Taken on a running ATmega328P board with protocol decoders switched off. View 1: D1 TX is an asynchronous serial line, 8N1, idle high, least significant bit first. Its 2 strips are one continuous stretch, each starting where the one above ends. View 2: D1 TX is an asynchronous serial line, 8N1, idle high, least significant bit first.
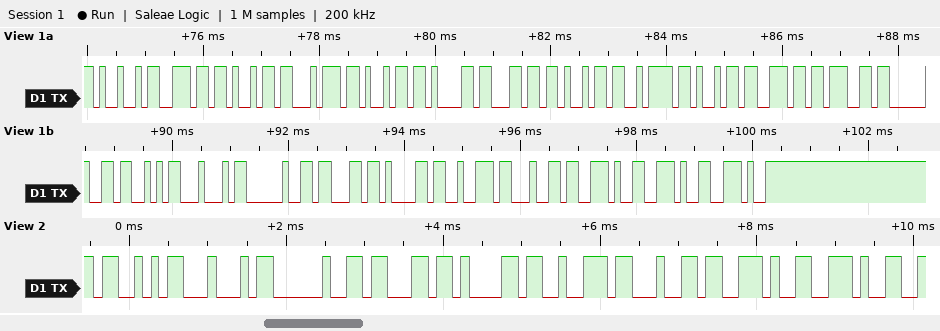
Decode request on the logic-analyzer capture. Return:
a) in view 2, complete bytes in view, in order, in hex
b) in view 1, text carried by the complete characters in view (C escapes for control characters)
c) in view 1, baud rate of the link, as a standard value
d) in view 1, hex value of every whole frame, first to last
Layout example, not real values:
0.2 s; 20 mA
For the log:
0x53 0x44 0x20 0x63 0x61 0x72 0x64 0x2E 0x2E; "Initializing SD card..."; 9600 baud; 0x49 0x6E 0x69 0x74 0x69 0x61 0x6C 0x69 0x7A 0x69 0x6E 0x67 0x20 0x53 0x44 0x20 0x63 0x61 0x72 0x64 0x2E 0x2E 0x2E
